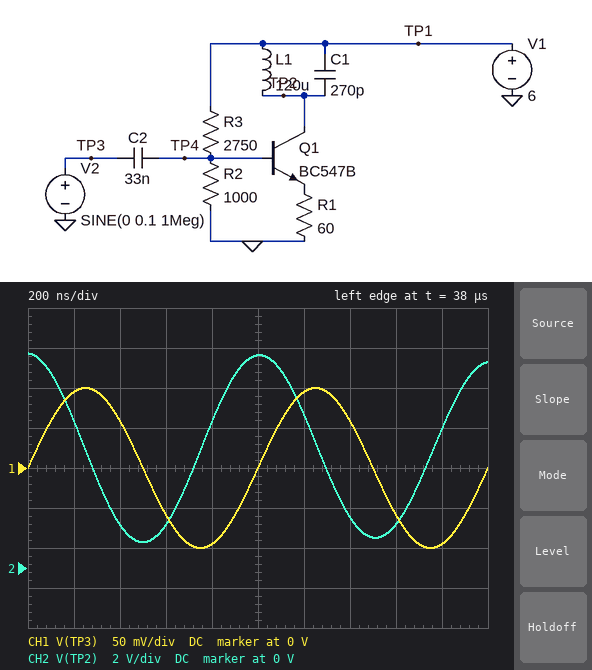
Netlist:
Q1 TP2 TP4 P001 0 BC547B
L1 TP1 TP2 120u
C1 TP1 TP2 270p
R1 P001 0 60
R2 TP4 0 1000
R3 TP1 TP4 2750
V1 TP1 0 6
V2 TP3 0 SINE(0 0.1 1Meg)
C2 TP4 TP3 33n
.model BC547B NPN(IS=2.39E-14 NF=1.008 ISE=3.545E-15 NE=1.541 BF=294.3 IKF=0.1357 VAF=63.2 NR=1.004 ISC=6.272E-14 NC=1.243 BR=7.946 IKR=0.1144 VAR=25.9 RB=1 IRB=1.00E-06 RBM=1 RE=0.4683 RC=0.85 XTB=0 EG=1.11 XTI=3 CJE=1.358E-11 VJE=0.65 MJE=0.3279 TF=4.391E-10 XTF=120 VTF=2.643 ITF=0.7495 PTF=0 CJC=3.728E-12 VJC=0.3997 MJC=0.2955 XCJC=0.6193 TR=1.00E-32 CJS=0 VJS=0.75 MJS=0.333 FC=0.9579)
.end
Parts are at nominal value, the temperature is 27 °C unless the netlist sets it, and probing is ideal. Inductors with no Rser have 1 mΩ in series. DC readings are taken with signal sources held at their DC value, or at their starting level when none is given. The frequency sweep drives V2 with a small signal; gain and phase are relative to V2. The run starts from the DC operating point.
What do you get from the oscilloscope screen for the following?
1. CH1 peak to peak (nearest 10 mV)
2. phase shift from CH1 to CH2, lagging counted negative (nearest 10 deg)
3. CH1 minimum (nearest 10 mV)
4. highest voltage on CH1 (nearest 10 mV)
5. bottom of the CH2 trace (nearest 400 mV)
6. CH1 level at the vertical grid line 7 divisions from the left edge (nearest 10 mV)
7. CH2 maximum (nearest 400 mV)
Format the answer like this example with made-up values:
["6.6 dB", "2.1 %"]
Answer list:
["200 mV", "90 deg", "-100 mV", "100 mV", "1.2 V", "60 mV", "10.8 V"]
